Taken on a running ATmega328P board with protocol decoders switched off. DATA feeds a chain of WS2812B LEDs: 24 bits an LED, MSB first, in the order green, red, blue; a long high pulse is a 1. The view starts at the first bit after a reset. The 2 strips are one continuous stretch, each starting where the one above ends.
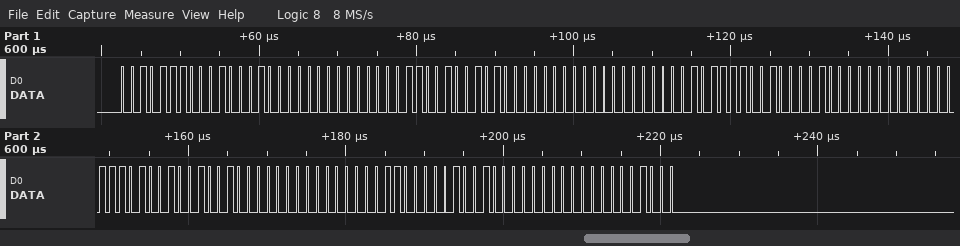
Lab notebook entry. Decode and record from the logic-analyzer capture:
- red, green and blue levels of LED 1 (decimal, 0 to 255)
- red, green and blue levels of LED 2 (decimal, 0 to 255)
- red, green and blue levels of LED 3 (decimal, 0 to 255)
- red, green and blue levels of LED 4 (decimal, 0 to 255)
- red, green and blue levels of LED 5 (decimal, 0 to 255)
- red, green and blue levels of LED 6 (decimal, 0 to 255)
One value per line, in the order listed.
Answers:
34, 46, 0
74, 6, 0
47, 0, 33
7, 0, 73
0, 32, 48
0, 72, 8
